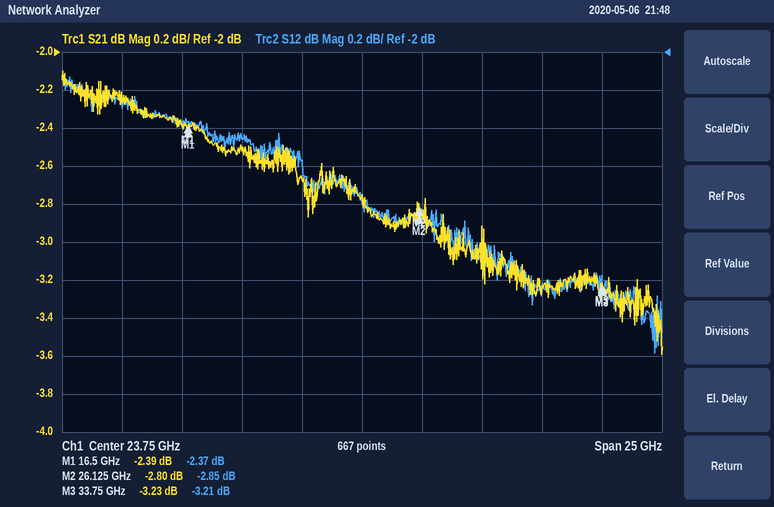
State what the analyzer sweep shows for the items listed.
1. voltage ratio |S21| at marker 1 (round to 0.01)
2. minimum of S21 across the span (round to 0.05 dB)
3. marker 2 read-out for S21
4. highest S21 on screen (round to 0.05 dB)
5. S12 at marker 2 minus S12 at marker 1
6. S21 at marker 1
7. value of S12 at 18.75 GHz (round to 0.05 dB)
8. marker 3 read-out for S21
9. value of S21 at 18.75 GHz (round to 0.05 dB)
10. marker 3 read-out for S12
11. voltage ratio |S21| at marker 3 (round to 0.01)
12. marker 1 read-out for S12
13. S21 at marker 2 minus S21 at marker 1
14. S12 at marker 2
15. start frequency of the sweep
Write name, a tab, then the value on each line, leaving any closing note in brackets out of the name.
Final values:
voltage ratio |S21| at marker 1	0.76
minimum of S21 across the span	-3.60 dB
marker 2 read-out for S21	-2.80 dB
highest S21 on screen	-2.10 dB
S12 at marker 2 minus S12 at marker 1	-0.48 dB
S21 at marker 1	-2.39 dB
value of S12 at 18.75 GHz	-2.45 dB
marker 3 read-out for S21	-3.23 dB
value of S21 at 18.75 GHz	-2.50 dB
marker 3 read-out for S12	-3.21 dB
voltage ratio |S21| at marker 3	0.69
marker 1 read-out for S12	-2.37 dB
S21 at marker 2 minus S21 at marker 1	-0.41 dB
S12 at marker 2	-2.85 dB
start frequency of the sweep	11.25 GHz
